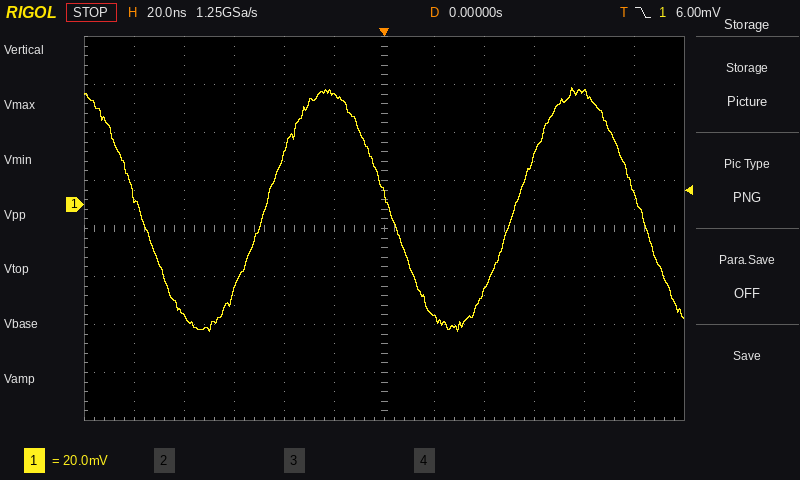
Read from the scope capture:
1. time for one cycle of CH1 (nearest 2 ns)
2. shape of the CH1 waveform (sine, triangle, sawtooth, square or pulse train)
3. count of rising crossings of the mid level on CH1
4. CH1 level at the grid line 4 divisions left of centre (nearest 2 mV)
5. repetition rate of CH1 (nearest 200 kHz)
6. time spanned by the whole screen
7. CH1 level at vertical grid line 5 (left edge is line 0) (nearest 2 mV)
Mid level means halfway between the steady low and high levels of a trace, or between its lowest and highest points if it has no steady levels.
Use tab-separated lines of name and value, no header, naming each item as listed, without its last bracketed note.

time for one cycle of CH1	100 ns
shape of the CH1 waveform	sine
count of rising crossings of the mid level on CH1	2
CH1 level at the grid line 4 divisions left of centre	-46 mV
repetition rate of CH1	10.0 MHz
time spanned by the whole screen	240 ns
CH1 level at vertical grid line 5 (left edge is line 0)	46 mV
